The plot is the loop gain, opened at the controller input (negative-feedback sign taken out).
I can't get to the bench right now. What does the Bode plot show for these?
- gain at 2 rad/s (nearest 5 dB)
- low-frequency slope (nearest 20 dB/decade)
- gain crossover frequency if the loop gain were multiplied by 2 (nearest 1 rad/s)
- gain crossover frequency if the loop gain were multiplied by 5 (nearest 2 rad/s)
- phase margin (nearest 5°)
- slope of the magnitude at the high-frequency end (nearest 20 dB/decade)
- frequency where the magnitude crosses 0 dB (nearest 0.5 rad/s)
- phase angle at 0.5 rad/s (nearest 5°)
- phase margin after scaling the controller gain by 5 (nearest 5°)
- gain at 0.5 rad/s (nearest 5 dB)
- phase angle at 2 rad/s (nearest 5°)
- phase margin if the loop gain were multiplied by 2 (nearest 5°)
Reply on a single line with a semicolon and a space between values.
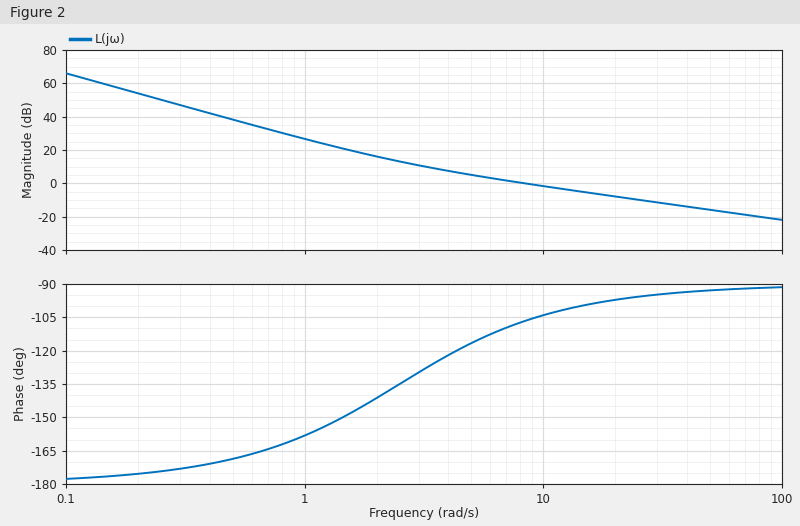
15 dB; -40 dB/decade; 16 rad/s; 40 rad/s; 75°; -20 dB/decade; 8.5 rad/s; -170°; 85°; 40 dB; -140°; 80°
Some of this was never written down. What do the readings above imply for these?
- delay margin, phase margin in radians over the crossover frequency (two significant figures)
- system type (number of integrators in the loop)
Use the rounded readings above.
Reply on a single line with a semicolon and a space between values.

0.15 s; 2
